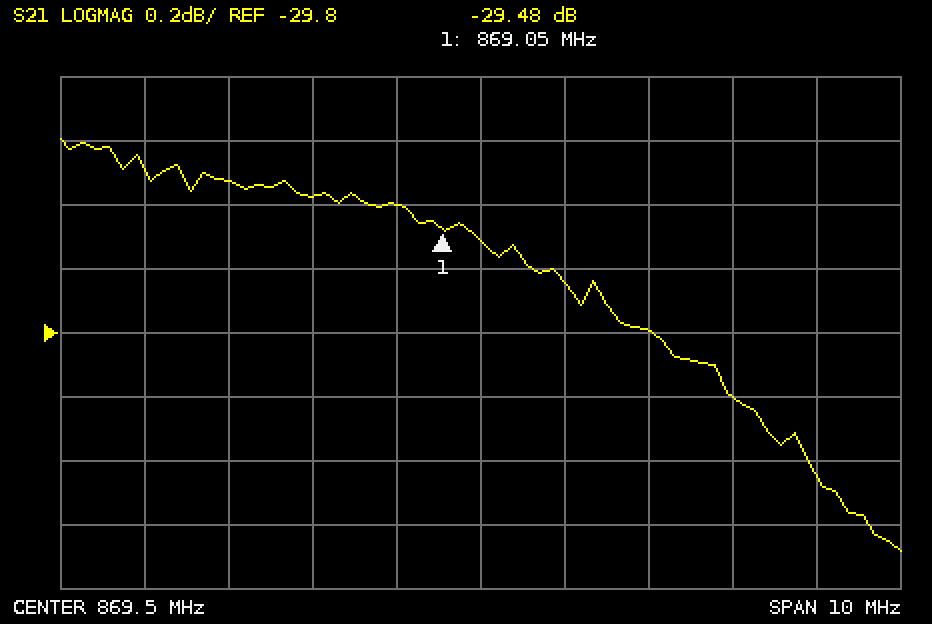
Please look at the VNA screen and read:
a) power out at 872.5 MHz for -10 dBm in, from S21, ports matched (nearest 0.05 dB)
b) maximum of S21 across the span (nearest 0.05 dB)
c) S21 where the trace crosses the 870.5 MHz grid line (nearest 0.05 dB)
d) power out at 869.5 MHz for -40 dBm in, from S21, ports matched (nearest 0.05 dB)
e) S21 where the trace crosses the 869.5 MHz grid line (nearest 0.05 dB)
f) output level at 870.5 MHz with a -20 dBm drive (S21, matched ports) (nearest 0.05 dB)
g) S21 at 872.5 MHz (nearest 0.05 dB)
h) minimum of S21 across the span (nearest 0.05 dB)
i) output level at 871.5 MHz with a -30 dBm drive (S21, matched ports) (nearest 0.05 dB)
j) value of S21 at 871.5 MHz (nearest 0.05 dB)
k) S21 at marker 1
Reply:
-40.00 dBm
-29.20 dB
-29.65 dB
-69.50 dBm
-29.50 dB
-49.65 dBm
-30.00 dB
-30.50 dB
-59.80 dBm
-29.80 dB
-29.48 dB
